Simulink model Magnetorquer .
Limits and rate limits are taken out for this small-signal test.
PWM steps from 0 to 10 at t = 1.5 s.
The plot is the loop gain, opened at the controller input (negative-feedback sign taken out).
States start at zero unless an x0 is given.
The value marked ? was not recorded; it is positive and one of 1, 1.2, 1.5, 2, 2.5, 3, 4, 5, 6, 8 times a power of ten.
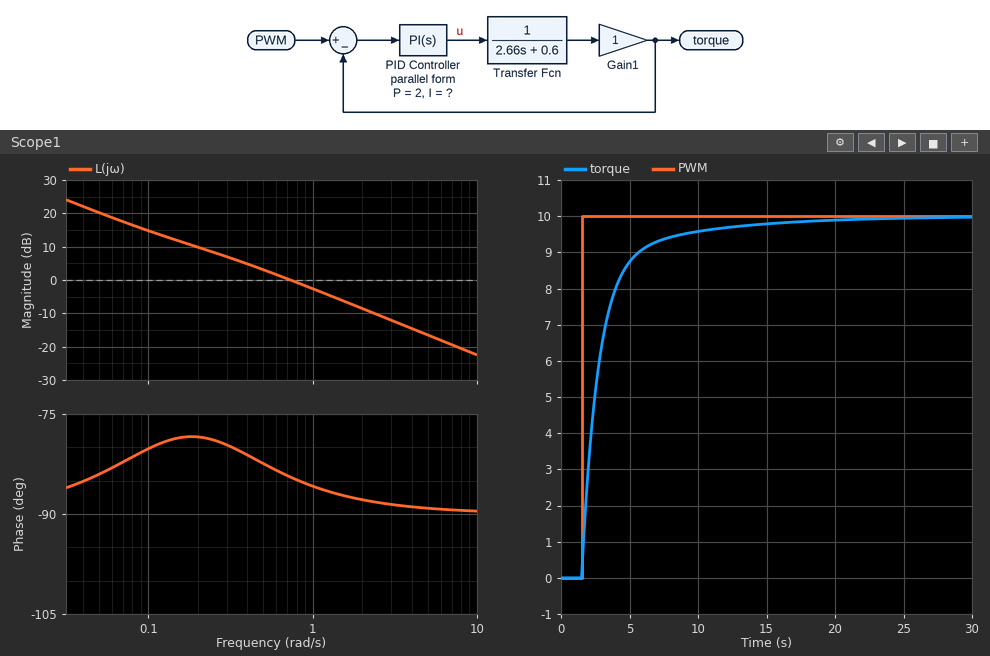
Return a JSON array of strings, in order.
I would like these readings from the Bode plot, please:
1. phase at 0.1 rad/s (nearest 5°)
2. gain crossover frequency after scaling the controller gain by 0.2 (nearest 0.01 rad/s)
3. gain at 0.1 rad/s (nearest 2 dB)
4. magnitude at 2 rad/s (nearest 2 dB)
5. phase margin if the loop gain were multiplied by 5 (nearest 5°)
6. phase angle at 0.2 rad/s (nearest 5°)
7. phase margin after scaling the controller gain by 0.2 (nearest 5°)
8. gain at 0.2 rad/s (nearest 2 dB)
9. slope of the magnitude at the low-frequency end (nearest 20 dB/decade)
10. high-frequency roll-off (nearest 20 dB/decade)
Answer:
["-80°", "0.11 rad/s", "14 dB", "-8 dB", "90°", "-80°", "100°", "10 dB", "-20 dB/decade", "-20 dB/decade"]
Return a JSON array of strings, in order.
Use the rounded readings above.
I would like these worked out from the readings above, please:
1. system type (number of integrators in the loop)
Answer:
["1"]
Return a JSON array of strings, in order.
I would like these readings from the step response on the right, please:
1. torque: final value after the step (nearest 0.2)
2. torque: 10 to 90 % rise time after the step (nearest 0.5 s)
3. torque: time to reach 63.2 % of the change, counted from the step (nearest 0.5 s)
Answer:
["10.0", "4.0 s", "1.5 s"]
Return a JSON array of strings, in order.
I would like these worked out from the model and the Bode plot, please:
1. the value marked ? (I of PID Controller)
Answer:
["0.3"]
